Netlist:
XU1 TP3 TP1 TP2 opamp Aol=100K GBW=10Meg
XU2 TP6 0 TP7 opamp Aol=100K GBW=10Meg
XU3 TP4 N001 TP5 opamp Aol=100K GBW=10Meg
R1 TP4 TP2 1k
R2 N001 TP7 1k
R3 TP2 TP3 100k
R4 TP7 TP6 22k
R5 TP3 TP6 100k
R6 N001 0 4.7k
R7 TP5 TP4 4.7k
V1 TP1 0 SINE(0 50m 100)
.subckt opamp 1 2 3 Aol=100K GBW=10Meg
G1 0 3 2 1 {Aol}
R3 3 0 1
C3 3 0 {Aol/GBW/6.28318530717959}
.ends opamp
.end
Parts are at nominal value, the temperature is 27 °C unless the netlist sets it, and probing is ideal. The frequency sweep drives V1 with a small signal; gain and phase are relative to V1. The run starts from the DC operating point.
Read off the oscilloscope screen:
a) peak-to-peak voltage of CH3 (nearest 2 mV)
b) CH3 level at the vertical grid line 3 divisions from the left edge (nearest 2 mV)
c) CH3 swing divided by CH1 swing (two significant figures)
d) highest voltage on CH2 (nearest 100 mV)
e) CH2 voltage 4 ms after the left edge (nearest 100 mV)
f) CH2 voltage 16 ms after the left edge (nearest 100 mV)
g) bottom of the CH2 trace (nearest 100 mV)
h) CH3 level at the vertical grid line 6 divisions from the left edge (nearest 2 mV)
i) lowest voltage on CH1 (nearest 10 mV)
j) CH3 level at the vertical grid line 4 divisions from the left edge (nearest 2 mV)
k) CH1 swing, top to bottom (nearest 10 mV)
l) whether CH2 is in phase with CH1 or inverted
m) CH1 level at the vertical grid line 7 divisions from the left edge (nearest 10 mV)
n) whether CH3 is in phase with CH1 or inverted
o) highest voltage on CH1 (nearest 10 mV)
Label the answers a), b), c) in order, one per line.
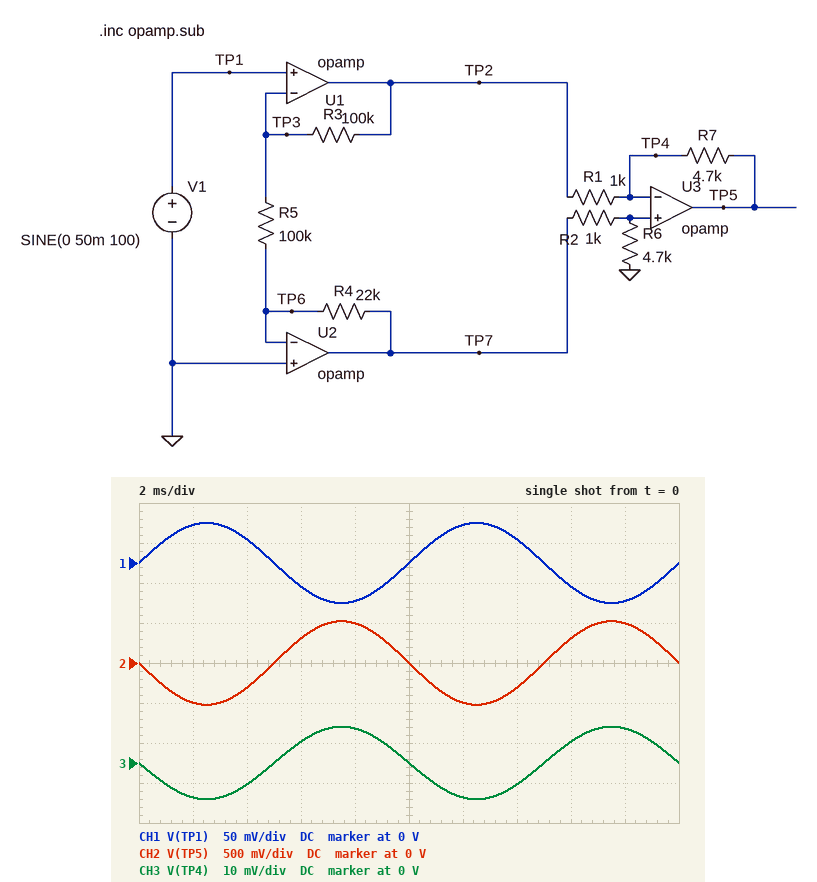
a) 18 mV
b) 6 mV
c) 0.18
d) 500 mV
e) -300 mV
f) 300 mV
g) -500 mV
h) -8 mV
i) -50 mV
j) 8 mV
k) 100 mV
l) inverted
m) 30 mV
n) inverted
o) 50 mV
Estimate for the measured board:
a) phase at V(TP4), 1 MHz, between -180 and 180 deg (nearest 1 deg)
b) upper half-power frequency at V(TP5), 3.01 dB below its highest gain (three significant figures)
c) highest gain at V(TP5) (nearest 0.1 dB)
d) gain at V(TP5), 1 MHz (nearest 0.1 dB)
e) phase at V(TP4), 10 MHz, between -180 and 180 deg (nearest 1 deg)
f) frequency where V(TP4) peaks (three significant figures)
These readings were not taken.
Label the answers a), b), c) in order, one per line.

a) 59 deg
b) 1.56 MHz
c) 20.4 dB
d) 18.9 dB
e) -52 deg
f) 2.84 MHz
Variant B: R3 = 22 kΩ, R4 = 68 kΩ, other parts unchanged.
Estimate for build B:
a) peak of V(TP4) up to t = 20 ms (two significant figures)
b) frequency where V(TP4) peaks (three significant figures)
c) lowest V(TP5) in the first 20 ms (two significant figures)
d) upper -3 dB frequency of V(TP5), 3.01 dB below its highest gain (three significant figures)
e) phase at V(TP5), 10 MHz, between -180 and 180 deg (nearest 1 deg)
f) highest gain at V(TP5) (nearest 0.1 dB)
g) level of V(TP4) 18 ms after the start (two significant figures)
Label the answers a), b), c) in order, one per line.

a) 28 mV
b) 2.98 MHz
c) -450 mV
d) 1.60 MHz
e) 38 deg
f) 19.0 dB
g) 27 mV
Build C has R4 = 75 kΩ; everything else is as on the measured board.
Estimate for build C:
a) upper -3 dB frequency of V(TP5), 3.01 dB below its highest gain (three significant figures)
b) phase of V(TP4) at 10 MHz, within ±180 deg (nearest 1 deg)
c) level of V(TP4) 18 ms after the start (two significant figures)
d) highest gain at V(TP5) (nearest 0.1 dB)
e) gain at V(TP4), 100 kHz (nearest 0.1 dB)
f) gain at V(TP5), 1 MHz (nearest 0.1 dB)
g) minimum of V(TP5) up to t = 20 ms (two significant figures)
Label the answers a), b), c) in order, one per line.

a) 1.48 MHz
b) -50 deg
c) 29 mV
d) 22.2 dB
e) -4.1 dB
f) 20.7 dB
g) -650 mV
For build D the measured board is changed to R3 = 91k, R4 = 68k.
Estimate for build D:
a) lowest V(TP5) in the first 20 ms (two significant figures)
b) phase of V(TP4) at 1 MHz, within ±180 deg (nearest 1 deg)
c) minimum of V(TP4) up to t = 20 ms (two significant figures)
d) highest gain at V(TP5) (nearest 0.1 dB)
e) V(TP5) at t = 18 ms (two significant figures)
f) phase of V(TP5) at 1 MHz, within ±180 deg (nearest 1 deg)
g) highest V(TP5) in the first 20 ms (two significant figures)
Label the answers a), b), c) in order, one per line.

a) -610 mV
b) 77 deg
c) -28 mV
d) 21.7 dB
e) 580 mV
f) 136 deg
g) 610 mV
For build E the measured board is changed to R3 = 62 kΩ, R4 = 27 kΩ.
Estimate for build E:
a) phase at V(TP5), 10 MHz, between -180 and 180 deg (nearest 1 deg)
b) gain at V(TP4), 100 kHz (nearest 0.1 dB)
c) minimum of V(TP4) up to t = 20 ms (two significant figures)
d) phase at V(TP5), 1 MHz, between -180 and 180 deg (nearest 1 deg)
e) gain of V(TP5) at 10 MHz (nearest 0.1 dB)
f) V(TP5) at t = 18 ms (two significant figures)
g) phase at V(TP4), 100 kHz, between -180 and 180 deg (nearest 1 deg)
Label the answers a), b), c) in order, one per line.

a) 38 deg
b) -12.6 dB
c) -11 mV
d) 140 deg
e) -2.9 dB
f) 420 mV
g) 156 deg
